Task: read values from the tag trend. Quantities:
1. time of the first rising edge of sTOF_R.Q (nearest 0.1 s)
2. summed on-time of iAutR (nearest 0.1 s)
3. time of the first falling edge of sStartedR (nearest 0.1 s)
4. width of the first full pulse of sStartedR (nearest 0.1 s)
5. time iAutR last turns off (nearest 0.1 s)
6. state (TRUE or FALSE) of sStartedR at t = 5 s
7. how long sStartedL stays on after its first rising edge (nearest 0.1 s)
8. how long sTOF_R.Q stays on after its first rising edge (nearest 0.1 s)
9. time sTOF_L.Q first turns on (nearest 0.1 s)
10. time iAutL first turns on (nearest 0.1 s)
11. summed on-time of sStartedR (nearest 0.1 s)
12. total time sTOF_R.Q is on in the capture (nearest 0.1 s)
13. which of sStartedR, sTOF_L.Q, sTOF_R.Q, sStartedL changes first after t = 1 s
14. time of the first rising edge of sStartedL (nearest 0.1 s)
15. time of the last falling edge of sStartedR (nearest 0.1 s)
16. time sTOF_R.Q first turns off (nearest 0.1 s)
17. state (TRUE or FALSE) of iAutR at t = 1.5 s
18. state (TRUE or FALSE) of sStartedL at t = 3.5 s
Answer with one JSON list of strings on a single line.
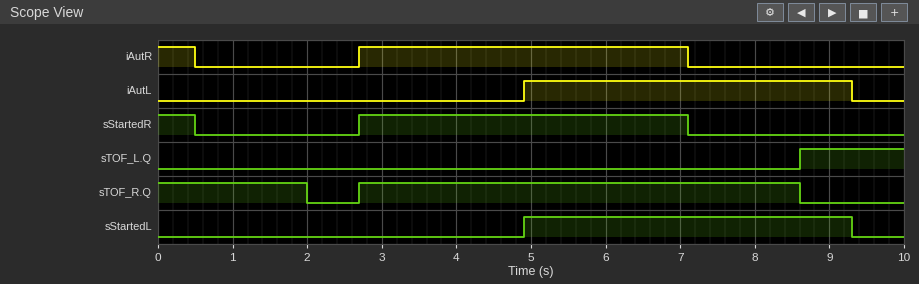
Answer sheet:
["2.7 s", "4.9 s", "0.5 s", "4.4 s", "7.1 s", "TRUE", "4.4 s", "5.9 s", "8.6 s", "4.9 s", "4.9 s", "7.9 s", "sTOF_R.Q", "4.9 s", "7.1 s", "2.0 s", "FALSE", "FALSE"]
